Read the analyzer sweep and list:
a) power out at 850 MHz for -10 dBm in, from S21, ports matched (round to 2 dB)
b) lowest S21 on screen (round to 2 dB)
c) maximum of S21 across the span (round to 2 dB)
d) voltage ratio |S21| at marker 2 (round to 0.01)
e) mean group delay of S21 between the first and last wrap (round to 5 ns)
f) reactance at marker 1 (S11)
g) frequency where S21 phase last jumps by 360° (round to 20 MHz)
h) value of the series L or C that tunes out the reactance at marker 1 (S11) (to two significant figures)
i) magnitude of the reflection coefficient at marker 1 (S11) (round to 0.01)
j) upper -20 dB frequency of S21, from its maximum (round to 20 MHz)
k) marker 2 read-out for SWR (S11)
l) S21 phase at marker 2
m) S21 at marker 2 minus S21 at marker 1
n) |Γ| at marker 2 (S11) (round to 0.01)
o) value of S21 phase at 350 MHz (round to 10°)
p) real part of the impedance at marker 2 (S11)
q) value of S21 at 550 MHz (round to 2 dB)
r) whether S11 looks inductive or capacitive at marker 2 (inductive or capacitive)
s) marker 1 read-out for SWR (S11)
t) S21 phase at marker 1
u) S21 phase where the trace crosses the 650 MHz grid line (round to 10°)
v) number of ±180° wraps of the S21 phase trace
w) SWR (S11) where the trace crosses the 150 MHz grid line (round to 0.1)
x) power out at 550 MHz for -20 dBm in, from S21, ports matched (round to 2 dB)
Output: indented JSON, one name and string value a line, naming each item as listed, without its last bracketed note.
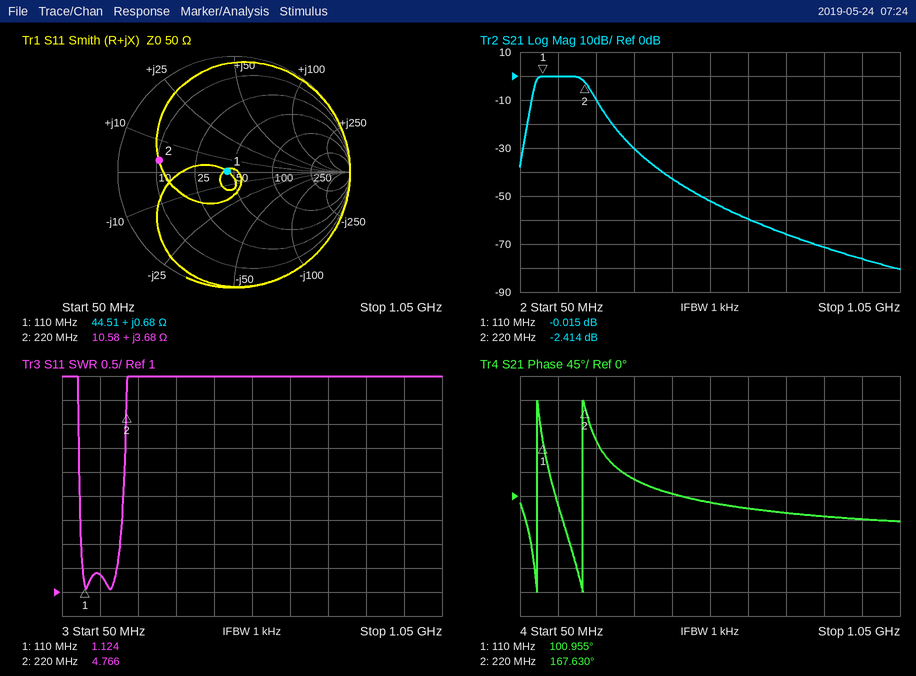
{
  "power out at 850 MHz for -10 dBm in, from S21, ports matched": "-82 dBm",
  "lowest S21 on screen": "-80 dB",
  "maximum of S21 across the span": "0 dB",
  "voltage ratio |S21| at marker 2": "0.76",
  "mean group delay of S21 between the first and last wrap": "10 ns",
  "reactance at marker 1": "+0.68 Ω",
  "frequency where S21 phase last jumps by 360°": "220 MHz",
  "value of the series L or C that tunes out the reactance at marker 1 (S11)": "2.1 nF",
  "magnitude of the reflection coefficient at marker 1 (S11)": "0.06",
  "upper -20 dB frequency of S21, from its maximum": "300 MHz",
  "marker 2 read-out for SWR": "4.766",
  "S21 phase at marker 2": "167.630°",
  "S21 at marker 2 minus S21 at marker 1": "-2.399 dB",
  "|Γ| at marker 2 (S11)": "0.65",
  "value of S21 phase at 350 MHz": "30°",
  "real part of the impedance at marker 2": "10.58 Ω",
  "value of S21 at 550 MHz": "-52 dB",
  "whether S11 looks inductive or capacitive at marker 2": "inductive",
  "marker 1 read-out for SWR": "1.124",
  "S21 phase at marker 1": "100.955°",
  "S21 phase where the trace crosses the 650 MHz grid line": "-20°",
  "number of ±180° wraps of the S21 phase trace": "2",
  "SWR (S11) where the trace crosses the 150 MHz grid line": "1.4",
  "power out at 550 MHz for -20 dBm in, from S21, ports matched": "-72 dBm"
}
